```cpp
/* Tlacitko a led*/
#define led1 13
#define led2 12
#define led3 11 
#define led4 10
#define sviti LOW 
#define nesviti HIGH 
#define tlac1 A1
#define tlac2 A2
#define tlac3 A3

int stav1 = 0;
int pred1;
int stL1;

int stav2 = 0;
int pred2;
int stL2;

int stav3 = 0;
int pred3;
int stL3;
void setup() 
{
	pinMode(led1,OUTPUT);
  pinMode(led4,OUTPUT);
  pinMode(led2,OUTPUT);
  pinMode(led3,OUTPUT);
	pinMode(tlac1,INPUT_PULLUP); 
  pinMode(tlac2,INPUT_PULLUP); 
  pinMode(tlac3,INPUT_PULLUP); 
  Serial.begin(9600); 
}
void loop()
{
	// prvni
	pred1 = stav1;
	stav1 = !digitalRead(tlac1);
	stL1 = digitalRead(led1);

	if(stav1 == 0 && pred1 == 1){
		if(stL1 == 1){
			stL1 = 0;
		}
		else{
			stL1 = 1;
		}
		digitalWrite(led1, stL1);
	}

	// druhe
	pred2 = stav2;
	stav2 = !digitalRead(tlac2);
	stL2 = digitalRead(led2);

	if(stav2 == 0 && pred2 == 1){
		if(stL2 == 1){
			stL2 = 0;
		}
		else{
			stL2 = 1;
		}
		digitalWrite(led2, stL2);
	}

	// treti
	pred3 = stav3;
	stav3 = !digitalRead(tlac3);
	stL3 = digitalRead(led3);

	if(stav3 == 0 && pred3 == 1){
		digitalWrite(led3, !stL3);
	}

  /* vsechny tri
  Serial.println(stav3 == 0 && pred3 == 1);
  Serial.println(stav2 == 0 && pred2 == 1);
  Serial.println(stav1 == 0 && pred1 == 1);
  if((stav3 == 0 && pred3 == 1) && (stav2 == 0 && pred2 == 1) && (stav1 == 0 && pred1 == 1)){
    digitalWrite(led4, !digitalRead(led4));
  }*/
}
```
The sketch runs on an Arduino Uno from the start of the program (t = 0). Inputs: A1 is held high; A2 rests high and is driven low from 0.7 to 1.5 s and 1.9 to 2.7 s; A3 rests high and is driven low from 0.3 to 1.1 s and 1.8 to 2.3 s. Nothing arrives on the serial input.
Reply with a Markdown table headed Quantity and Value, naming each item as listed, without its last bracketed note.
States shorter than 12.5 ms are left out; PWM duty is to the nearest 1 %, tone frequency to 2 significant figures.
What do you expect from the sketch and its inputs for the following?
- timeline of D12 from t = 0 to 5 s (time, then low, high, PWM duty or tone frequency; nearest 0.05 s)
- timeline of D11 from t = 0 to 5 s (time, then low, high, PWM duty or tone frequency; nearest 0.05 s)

| Quantity | Value |
|---|---|
| timeline of D12 from t = 0 to 5 s | 0 s low; 1.5 s high; 2.7 s low |
| timeline of D11 from t = 0 to 5 s | 0 s low; 1.1 s high; 2.3 s low |
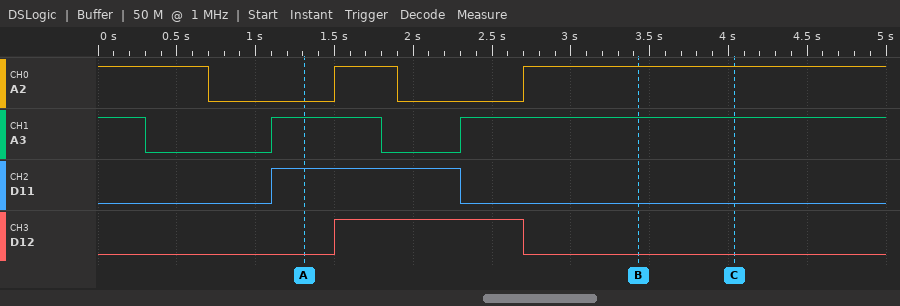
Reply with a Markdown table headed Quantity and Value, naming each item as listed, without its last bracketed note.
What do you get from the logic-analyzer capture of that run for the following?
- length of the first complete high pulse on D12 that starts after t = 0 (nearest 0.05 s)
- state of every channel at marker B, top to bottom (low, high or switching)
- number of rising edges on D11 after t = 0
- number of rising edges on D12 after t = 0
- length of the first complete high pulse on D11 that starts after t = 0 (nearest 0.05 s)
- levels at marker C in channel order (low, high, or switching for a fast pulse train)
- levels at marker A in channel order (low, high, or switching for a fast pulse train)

| Quantity | Value |
|---|---|
| length of the first complete high pulse on D12 that starts after t = 0 | 1.20 s |
| state of every channel at marker B, top to bottom | A2 high, A3 high, D11 low, D12 low |
| number of rising edges on D11 after t = 0 | 1 |
| number of rising edges on D12 after t = 0 | 1 |
| length of the first complete high pulse on D11 that starts after t = 0 | 1.20 s |
| levels at marker C in channel order | A2 high, A3 high, D11 low, D12 low |
| levels at marker A in channel order | A2 low, A3 high, D11 high, D12 low |
